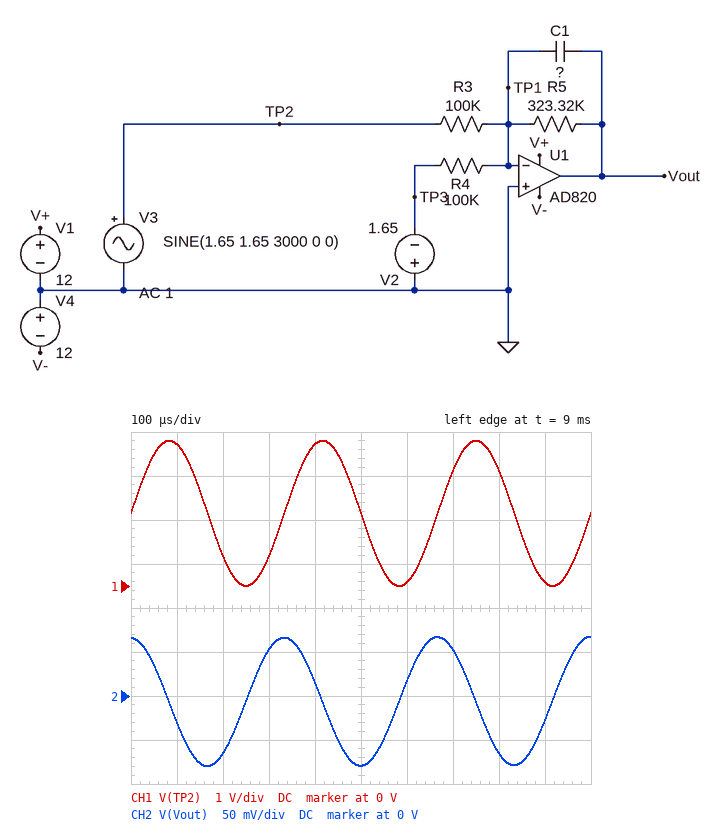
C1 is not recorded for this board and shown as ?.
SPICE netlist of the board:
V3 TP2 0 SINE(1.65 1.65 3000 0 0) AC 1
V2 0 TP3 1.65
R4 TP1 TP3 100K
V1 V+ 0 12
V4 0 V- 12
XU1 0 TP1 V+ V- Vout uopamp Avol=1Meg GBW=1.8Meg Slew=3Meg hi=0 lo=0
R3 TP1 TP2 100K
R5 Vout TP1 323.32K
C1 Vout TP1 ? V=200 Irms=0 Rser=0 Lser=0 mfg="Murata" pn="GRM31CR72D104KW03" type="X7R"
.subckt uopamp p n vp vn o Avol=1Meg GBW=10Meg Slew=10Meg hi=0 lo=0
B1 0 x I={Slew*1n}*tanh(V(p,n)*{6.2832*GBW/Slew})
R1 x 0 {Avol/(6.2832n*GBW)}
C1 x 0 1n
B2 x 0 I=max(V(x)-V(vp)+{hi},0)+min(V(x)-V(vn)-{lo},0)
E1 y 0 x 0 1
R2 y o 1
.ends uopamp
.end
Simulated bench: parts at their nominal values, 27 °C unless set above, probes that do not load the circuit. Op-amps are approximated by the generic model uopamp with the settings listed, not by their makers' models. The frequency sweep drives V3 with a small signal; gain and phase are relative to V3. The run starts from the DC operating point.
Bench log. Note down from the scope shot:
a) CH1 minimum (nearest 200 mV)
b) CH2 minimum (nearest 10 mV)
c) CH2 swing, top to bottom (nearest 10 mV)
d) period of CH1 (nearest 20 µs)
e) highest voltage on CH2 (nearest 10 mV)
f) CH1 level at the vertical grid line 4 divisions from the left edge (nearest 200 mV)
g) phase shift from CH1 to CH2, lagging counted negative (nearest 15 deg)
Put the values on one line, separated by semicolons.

0 V; -80 mV; 150 mV; 340 µs; 70 mV; 3.2 V; 90 deg
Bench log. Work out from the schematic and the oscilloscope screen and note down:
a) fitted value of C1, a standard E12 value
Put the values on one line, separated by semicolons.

12 nF
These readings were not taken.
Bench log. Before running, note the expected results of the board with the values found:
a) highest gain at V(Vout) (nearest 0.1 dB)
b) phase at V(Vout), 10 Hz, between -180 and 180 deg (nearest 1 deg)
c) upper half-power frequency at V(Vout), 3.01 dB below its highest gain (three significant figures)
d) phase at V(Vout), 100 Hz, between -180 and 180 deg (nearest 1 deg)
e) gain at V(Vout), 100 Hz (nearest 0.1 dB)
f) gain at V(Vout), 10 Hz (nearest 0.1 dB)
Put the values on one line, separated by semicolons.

10.2 dB; 166 deg; 41.0 Hz; 112 deg; 1.8 dB; 9.9 dB
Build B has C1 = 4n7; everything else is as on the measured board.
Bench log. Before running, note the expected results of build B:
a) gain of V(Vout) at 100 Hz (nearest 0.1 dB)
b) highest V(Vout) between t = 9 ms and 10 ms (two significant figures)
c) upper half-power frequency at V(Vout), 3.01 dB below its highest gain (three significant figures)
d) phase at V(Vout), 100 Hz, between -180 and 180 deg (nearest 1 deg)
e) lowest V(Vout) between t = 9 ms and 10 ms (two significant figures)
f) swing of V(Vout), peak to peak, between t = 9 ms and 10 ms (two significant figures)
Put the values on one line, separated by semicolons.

7.4 dB; 190 mV; 105 Hz; 136 deg; -190 mV; 370 mV
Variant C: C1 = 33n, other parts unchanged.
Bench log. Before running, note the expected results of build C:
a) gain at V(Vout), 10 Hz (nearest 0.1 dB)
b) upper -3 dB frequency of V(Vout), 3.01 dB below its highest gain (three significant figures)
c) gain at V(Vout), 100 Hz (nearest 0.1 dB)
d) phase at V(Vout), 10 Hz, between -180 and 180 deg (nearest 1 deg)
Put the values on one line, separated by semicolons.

8.6 dB; 14.9 Hz; -6.4 dB; 146 deg
